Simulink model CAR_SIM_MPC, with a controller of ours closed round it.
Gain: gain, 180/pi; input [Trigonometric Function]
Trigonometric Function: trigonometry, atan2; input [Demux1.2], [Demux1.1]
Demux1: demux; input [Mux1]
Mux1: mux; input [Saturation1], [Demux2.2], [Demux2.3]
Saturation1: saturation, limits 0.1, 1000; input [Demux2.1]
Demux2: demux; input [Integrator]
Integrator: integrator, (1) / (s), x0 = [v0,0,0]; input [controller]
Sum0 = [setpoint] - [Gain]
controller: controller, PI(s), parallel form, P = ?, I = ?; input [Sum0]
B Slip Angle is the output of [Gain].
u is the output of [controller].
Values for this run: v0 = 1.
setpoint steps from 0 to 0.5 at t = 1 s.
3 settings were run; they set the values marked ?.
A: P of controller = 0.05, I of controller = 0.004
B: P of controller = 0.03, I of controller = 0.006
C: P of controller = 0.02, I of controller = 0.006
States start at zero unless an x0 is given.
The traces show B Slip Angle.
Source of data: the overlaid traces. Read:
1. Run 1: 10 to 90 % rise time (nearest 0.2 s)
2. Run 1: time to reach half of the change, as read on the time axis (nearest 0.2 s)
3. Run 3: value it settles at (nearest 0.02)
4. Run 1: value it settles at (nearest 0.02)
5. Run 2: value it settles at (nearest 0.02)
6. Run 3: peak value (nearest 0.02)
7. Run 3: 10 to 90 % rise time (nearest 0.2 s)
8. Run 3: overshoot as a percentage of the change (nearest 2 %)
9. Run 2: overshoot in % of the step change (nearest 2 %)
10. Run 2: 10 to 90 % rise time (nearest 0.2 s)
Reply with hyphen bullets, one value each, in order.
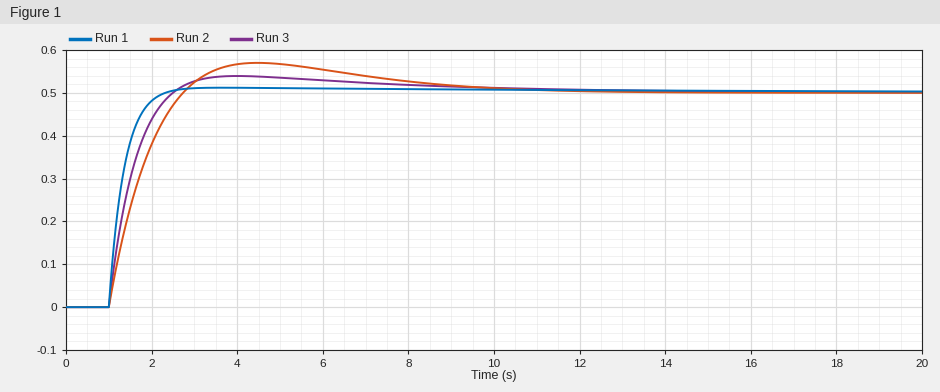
- 0.8 s
- 1.2 s
- 0.50
- 0.50
- 0.50
- 0.54
- 1.0 s
- 8 %
- 14 %
- 1.2 s
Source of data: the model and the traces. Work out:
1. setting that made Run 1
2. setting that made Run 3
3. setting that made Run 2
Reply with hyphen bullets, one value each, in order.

- A
- B
- C
